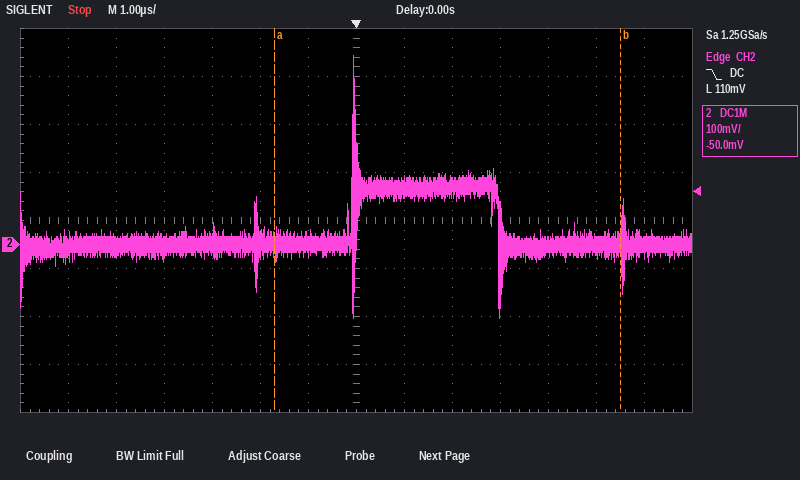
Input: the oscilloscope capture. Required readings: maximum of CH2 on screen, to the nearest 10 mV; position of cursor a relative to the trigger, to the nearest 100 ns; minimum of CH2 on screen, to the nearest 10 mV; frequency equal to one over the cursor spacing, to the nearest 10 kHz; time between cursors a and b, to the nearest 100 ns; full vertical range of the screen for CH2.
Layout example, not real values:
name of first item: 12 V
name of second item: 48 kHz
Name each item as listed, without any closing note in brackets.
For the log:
maximum of CH2 on screen, to the nearest 10 mV: 390 mV
position of cursor a relative to the trigger, to the nearest 100 ns: -1.7 µs
minimum of CH2 on screen, to the nearest 10 mV: -150 mV
frequency equal to one over the cursor spacing, to the nearest 10 kHz: 140 kHz
time between cursors a and b, to the nearest 100 ns: 7.2 µs
full vertical range of the screen for CH2: 800 mV
